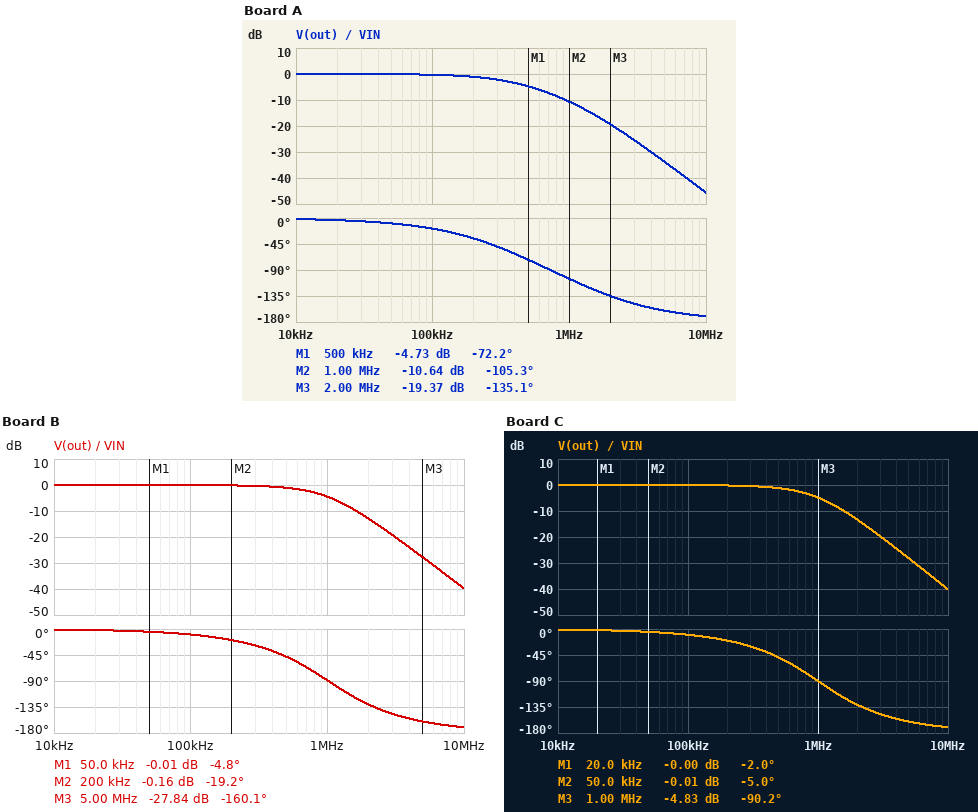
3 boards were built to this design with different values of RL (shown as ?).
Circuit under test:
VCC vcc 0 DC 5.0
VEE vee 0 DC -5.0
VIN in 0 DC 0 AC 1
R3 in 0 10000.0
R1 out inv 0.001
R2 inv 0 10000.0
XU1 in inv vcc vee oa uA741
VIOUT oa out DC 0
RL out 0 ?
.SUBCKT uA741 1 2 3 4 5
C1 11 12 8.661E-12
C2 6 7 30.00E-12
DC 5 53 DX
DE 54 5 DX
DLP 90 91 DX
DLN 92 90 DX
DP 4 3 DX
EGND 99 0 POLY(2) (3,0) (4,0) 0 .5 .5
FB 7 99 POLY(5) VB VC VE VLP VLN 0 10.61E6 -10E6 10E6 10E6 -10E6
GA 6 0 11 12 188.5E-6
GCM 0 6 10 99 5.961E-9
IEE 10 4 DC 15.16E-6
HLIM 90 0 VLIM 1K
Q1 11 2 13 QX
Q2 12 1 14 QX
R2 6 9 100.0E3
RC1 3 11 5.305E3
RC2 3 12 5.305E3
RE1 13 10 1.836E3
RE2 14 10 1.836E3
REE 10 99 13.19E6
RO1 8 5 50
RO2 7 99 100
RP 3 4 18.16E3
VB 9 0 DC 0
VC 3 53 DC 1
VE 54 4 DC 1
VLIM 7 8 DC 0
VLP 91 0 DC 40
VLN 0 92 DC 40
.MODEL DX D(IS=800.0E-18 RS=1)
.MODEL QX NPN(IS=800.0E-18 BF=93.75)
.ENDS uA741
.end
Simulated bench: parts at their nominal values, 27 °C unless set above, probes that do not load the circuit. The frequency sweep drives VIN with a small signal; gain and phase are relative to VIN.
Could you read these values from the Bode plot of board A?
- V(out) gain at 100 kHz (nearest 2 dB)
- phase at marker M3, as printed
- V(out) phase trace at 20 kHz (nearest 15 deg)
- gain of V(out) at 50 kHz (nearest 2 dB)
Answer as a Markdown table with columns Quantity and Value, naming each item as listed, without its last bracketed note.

| Quantity | Value |
|---|---|
| V(out) gain at 100 kHz | 0 dB |
| phase at marker M3, as printed | -135.1 deg |
| V(out) phase trace at 20 kHz | 0 deg |
| gain of V(out) at 50 kHz | 0 dB |
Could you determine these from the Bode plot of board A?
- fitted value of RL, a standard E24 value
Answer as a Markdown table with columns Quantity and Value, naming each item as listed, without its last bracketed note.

| Quantity | Value |
|---|---|
| fitted value of RL, a standard E24 value | 22 Ω |
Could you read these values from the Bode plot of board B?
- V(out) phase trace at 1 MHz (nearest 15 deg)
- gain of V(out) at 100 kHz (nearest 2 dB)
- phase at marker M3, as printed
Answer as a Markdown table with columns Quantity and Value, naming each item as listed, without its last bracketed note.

| Quantity | Value |
|---|---|
| V(out) phase trace at 1 MHz | -90 deg |
| gain of V(out) at 100 kHz | 0 dB |
| phase at marker M3, as printed | -160.1 deg |
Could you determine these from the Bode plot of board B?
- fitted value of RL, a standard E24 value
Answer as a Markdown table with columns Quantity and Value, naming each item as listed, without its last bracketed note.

| Quantity | Value |
|---|---|
| fitted value of RL, a standard E24 value | 75 Ω |
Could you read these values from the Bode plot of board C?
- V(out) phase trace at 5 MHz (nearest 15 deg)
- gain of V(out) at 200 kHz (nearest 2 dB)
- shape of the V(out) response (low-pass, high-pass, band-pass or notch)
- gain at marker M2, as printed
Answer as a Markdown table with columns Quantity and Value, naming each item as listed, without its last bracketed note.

| Quantity | Value |
|---|---|
| V(out) phase trace at 5 MHz | -165 deg |
| gain of V(out) at 200 kHz | 0 dB |
| shape of the V(out) response | low-pass |
| gain at marker M2, as printed | -0.01 dB |
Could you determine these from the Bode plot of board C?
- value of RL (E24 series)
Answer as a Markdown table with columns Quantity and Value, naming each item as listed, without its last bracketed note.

| Quantity | Value |
|---|---|
| value of RL | 68 Ω |
